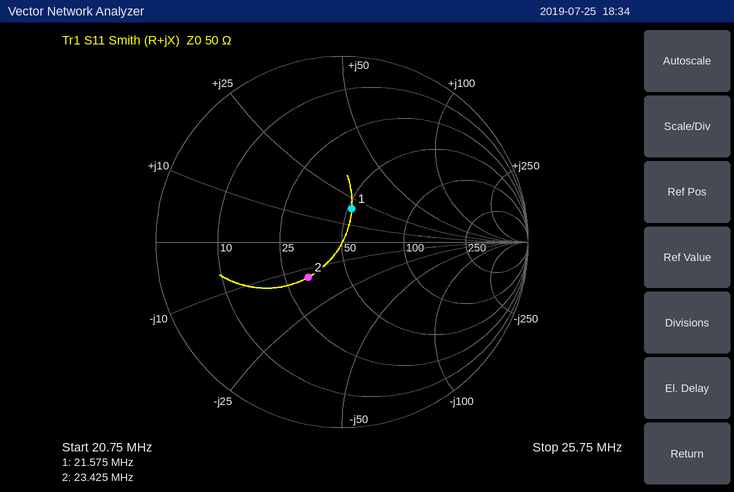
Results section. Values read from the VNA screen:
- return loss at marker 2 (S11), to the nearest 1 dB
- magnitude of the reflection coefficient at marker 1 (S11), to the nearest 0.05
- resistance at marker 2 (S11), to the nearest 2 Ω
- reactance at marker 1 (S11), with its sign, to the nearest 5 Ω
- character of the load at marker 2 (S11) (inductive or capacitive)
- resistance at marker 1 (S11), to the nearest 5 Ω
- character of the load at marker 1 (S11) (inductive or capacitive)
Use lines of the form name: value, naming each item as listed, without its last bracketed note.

return loss at marker 2 (S11), to the nearest 1 dB: 12 dB
magnitude of the reflection coefficient at marker 1 (S11), to the nearest 0.05: 0.20
resistance at marker 2 (S11), to the nearest 2 Ω: 32 Ω
reactance at marker 1 (S11), with its sign, to the nearest 5 Ω: +20 Ω
character of the load at marker 2 (S11): capacitive
resistance at marker 1 (S11), to the nearest 5 Ω: 50 Ω
character of the load at marker 1 (S11): inductive
